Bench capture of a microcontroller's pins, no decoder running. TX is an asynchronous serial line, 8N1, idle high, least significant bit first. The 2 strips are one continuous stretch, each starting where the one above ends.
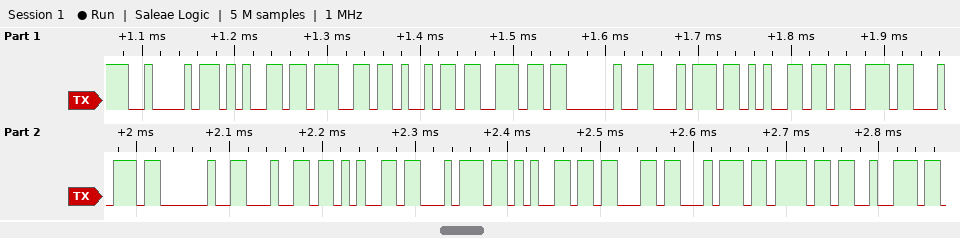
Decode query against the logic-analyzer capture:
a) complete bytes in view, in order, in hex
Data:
0x42 0x65 0x67 0x69 0x6E 0x20 0x74 0x65 0x73 0x74 0x20 0x64 0x65 0x74 0x65 0x63 0x74 0x6F 0x72
